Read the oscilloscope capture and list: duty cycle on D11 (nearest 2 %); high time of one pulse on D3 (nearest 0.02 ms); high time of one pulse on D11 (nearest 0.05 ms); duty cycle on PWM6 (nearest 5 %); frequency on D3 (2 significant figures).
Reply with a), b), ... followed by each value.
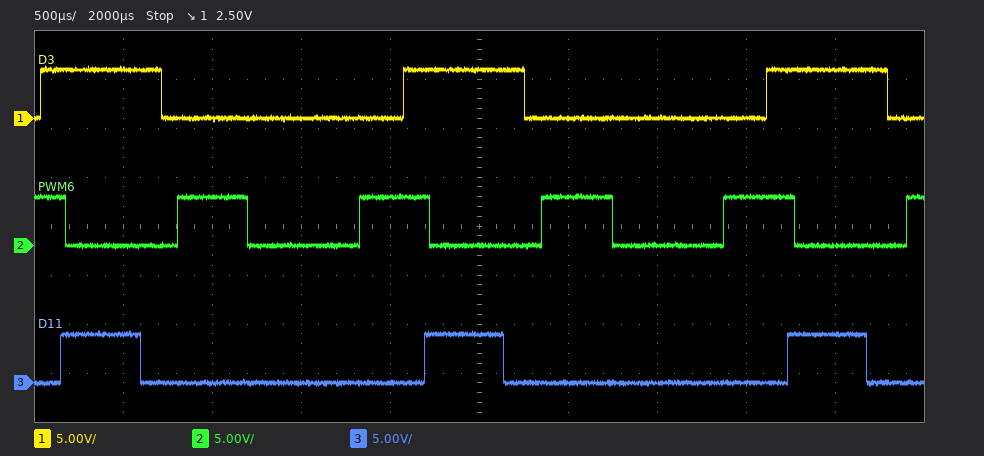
a) 22 %
b) 0.68 ms
c) 0.45 ms
d) 40 %
e) 490 Hz
